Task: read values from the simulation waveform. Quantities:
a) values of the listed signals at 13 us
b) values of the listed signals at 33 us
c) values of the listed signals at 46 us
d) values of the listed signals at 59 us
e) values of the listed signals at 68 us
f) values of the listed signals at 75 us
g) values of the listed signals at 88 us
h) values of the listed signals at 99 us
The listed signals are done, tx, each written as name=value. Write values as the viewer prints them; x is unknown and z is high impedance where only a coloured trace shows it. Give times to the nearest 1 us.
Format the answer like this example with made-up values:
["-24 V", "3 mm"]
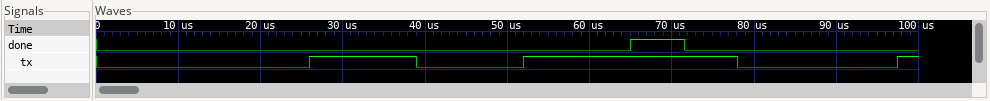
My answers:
["done=0, tx=0", "done=0, tx=1", "done=0, tx=0", "done=0, tx=1", "done=1, tx=1", "done=0, tx=1", "done=0, tx=0", "done=0, tx=1"]
